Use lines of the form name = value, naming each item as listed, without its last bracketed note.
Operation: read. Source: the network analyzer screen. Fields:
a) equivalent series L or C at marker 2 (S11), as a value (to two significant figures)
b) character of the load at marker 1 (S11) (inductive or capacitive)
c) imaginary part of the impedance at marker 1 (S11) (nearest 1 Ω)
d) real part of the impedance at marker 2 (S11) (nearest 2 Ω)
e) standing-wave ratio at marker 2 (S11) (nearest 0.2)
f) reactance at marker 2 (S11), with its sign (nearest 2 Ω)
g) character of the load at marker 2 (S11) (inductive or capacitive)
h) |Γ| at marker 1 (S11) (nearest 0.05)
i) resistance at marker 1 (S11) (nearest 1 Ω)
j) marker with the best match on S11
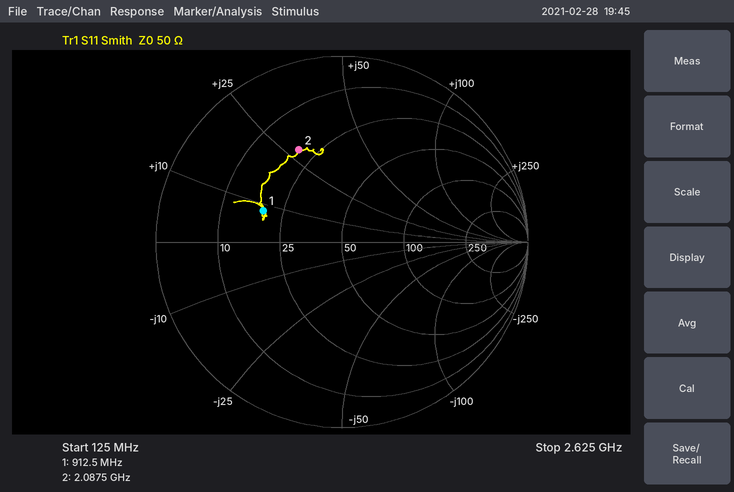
equivalent series L or C at marker 2 (S11), as a value = 2.1 nH
character of the load at marker 1 (S11) = inductive
imaginary part of the impedance at marker 1 (S11) = +8 Ω
real part of the impedance at marker 2 (S11) = 20 Ω
standing-wave ratio at marker 2 (S11) = 3.4
reactance at marker 2 (S11), with its sign = +28 Ω
character of the load at marker 2 (S11) = inductive
|Γ| at marker 1 (S11) = 0.45
resistance at marker 1 (S11) = 19 Ω
marker with the best match on S11 = marker 1
